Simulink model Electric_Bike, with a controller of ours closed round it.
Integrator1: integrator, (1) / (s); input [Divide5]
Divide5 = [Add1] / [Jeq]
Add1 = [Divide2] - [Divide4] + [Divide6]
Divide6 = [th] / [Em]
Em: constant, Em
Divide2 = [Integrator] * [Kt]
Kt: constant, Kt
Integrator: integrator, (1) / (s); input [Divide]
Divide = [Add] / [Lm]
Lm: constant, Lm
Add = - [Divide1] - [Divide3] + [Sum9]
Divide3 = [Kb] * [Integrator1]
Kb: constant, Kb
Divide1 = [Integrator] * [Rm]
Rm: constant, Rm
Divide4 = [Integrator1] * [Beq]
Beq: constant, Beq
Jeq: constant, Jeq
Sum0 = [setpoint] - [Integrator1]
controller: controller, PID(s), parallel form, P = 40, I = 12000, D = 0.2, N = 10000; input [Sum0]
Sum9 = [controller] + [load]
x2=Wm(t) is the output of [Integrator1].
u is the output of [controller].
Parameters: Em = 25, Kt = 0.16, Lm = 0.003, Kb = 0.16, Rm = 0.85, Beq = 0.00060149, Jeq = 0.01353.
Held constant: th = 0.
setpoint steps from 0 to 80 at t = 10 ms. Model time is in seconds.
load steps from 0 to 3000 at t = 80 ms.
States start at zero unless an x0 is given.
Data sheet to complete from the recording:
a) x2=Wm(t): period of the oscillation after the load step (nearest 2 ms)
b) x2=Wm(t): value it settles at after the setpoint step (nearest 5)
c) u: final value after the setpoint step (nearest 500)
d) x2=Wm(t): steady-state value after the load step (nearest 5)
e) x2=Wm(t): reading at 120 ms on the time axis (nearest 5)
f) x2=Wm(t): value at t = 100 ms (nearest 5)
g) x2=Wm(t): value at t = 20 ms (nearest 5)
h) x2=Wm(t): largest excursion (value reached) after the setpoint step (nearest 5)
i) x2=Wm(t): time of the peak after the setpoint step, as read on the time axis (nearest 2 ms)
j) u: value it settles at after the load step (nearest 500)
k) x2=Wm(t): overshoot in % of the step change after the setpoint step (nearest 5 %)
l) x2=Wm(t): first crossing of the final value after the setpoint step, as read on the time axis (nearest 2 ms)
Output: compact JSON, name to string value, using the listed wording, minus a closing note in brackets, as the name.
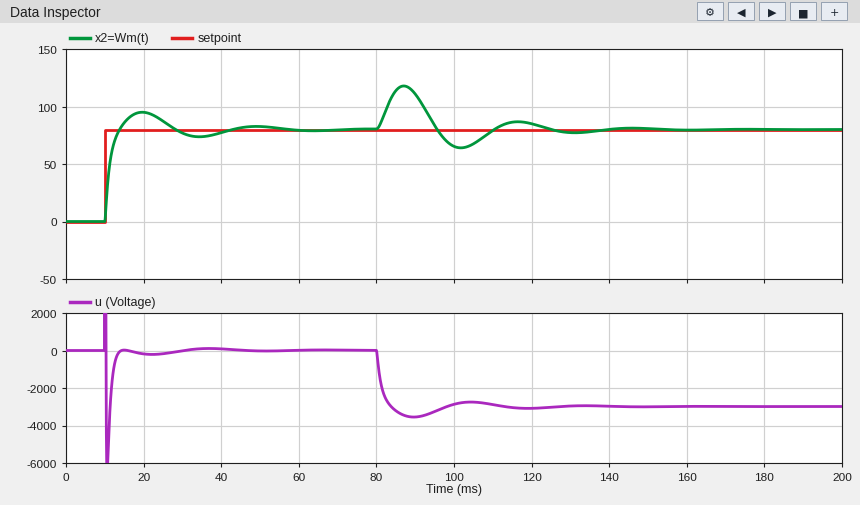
{"x2=Wm(t): period of the oscillation after the load step": "30 ms", "x2=Wm(t): value it settles at after the setpoint step": "80", "u: final value after the setpoint step": "0", "x2=Wm(t): steady-state value after the load step": "80", "x2=Wm(t): reading at 120 ms on the time axis": "85", "x2=Wm(t): value at t = 100 ms": "65", "x2=Wm(t): value at t = 20 ms": "95", "x2=Wm(t): largest excursion (value reached) after the setpoint step": "95", "x2=Wm(t): time of the peak after the setpoint step, as read on the time axis": "20 ms", "u: value it settles at after the load step": "-3000", "x2=Wm(t): overshoot in % of the step change after the setpoint step": "20 %", "x2=Wm(t): first crossing of the final value after the setpoint step, as read on the time axis": "14 ms"}
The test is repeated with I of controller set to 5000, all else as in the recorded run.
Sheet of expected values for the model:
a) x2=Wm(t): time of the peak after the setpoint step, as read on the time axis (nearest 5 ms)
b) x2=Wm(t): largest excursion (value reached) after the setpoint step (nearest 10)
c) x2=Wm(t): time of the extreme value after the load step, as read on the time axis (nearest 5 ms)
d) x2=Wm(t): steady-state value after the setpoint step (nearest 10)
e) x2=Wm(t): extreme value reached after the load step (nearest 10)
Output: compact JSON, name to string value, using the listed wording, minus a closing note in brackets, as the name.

{"x2=Wm(t): time of the peak after the setpoint step, as read on the time axis": "25 ms", "x2=Wm(t): largest excursion (value reached) after the setpoint step": "90", "x2=Wm(t): time of the extreme value after the load step, as read on the time axis": "90 ms", "x2=Wm(t): steady-state value after the setpoint step": "80", "x2=Wm(t): extreme value reached after the load step": "130"}
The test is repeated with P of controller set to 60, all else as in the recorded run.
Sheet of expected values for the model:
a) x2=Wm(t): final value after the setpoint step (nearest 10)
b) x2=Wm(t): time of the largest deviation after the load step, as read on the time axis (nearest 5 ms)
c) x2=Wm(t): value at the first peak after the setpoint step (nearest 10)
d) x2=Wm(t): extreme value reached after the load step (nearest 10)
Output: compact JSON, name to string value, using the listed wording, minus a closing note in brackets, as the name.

{"x2=Wm(t): final value after the setpoint step": "80", "x2=Wm(t): time of the largest deviation after the load step, as read on the time axis": "85 ms", "x2=Wm(t): value at the first peak after the setpoint step": "90", "x2=Wm(t): extreme value reached after the load step": "110"}
